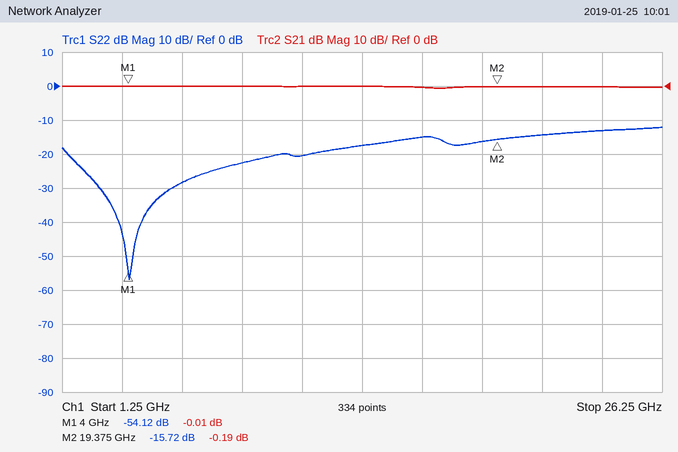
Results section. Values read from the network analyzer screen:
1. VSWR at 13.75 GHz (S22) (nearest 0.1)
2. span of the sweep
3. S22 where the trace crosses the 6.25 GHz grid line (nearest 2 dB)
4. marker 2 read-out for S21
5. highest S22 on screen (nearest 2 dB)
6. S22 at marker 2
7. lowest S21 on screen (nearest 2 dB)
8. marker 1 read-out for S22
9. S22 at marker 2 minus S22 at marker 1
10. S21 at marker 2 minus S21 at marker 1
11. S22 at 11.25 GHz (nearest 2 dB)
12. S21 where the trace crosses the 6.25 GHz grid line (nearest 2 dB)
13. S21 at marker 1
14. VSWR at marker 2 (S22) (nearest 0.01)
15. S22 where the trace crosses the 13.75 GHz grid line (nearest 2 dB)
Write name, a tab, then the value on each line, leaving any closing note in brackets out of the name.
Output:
VSWR at 13.75 GHz (S22)	1.3
span of the sweep	25 GHz
S22 where the trace crosses the 6.25 GHz grid line	-28 dB
marker 2 read-out for S21	-0.19 dB
highest S22 on screen	-12 dB
S22 at marker 2	-15.72 dB
lowest S21 on screen	0 dB
marker 1 read-out for S22	-54.12 dB
S22 at marker 2 minus S22 at marker 1	38.40 dB
S21 at marker 2 minus S21 at marker 1	-0.18 dB
S22 at 11.25 GHz	-20 dB
S21 where the trace crosses the 6.25 GHz grid line	0 dB
S21 at marker 1	-0.01 dB
VSWR at marker 2 (S22)	1.39
S22 where the trace crosses the 13.75 GHz grid line	-18 dB
